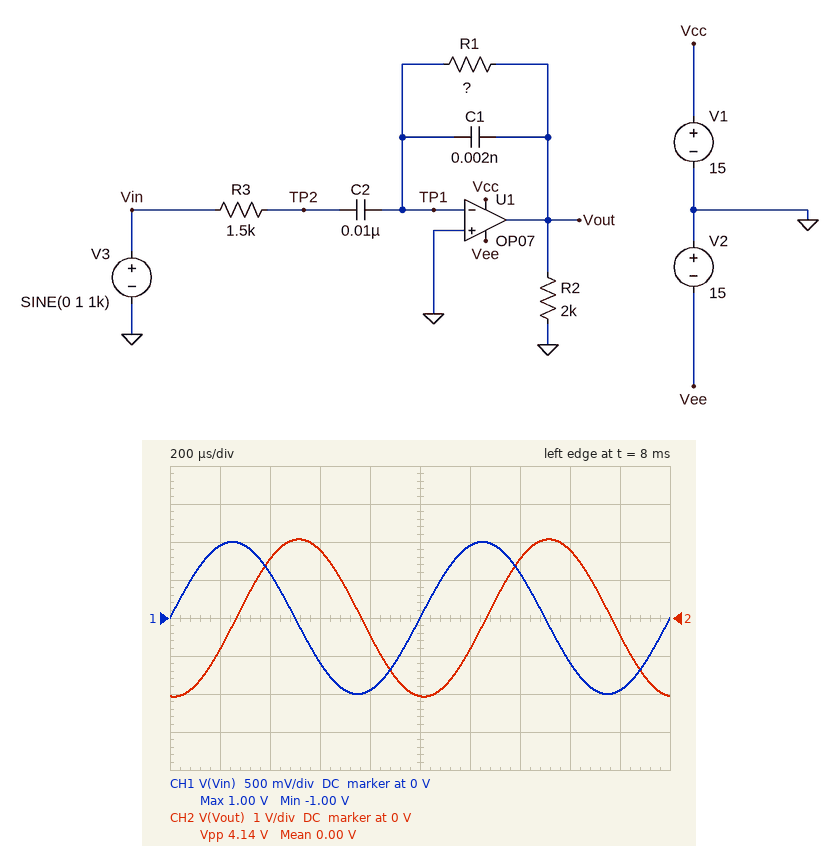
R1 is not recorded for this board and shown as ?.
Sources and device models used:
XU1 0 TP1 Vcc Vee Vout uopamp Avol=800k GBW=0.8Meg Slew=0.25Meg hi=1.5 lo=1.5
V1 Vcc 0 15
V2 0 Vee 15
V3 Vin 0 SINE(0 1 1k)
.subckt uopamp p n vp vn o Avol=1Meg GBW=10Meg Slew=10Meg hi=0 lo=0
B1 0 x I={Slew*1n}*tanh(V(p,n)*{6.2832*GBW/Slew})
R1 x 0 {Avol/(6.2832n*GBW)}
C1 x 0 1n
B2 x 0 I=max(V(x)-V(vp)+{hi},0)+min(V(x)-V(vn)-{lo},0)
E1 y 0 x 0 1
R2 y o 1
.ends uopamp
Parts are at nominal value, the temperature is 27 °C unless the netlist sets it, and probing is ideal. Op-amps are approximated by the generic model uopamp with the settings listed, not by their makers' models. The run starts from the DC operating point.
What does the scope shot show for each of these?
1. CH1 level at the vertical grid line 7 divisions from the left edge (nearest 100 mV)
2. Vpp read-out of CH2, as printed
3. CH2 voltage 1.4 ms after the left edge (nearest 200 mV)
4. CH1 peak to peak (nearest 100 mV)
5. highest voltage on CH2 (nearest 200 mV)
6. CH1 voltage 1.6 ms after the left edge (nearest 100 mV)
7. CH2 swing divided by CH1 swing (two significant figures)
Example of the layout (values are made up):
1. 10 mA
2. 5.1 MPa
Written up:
1. 600 mV
2. 4.14 V
3. 1.6 V
4. 2.0 V
5. 2.0 V
6. -600 mV
7. 2.1
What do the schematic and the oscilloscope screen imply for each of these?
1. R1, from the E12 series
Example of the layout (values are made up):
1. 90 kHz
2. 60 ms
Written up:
1. 33 kΩ
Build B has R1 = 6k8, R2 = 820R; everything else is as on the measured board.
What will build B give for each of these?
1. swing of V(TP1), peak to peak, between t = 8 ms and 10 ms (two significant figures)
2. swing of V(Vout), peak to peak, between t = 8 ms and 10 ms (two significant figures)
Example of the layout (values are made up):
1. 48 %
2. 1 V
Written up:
1. 1.1 mV
2. 850 mV
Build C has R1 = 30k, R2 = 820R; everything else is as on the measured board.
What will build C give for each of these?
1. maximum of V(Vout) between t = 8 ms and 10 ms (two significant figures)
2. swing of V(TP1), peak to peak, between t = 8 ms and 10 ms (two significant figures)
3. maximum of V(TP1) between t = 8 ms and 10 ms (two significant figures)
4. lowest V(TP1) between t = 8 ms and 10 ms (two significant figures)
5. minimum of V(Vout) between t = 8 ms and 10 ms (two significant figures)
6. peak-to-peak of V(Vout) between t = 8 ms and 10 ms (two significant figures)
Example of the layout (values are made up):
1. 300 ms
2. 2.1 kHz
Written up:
1. 1.9 V
2. 4.7 mV
3. 2.4 mV
4. -2.4 mV
5. -1.9 V
6. 3.8 V
